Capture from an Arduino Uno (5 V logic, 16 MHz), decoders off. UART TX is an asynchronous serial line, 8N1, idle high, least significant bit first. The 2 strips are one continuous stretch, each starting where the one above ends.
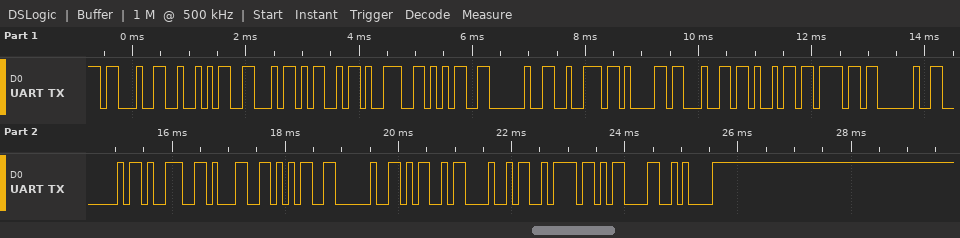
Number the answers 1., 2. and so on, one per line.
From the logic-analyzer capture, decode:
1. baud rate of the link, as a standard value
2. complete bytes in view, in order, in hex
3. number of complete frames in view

1. 9600 baud
2. 23 52 46 4D 39 35 20 72 61 64 69 6F 20 40 39 31 35 20 4D 48 7A 0D 0A
3. 23
